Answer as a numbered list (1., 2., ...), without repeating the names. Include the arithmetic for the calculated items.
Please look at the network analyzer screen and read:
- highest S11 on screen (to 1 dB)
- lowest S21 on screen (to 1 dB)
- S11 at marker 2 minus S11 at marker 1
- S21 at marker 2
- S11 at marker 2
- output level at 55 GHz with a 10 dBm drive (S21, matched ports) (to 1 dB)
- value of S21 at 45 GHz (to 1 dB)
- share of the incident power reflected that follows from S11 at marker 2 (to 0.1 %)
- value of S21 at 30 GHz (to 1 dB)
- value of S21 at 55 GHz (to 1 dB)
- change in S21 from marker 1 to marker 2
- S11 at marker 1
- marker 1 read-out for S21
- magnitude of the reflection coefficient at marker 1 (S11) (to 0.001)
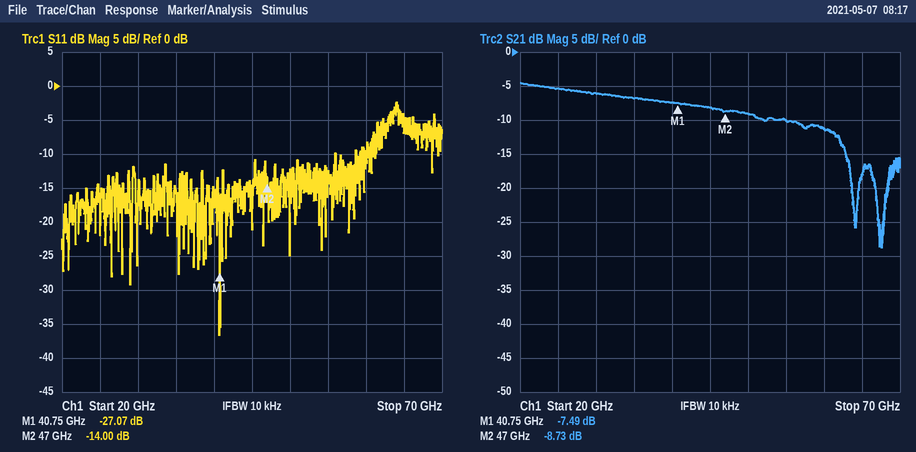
1. -2 dB
2. -29 dB
3. -14 − (-27.07) = 13.07 dB
4. -8.73 dB
5. -14.00 dB
6. 10 dBm + (-10 dB) = 0 dBm
7. -8 dB
8. 10^(-14/10) ≈ 4.0 %
9. -6 dB
10. -10 dB
11. -8.73 − (-7.49) = -1.24 dB
12. -27.07 dB
13. -7.49 dB
14. 10^(-27.07/20) ≈ 0.044
